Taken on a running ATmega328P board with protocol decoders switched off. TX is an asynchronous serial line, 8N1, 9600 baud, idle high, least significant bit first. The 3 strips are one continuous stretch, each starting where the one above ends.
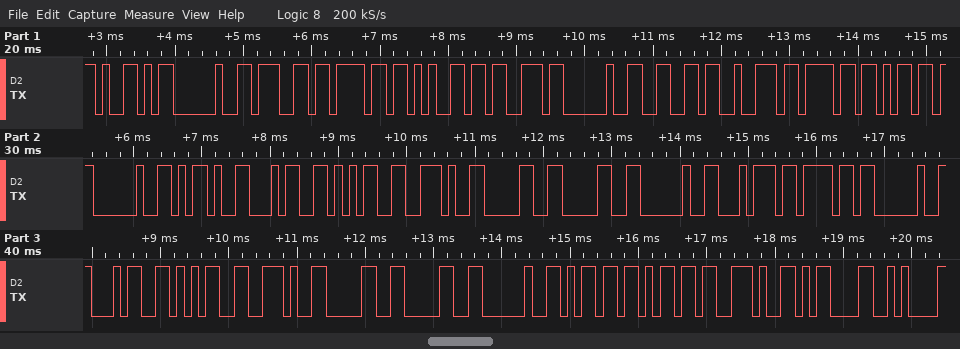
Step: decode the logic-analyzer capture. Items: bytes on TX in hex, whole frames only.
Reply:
59 20 67 6F 65 73 20 66 72 6F 6D 20 2D 34 35 2E 30 30 20 74 6F 20 34 35 2E 30 30 20 6D 6D 2E 0D 0A
